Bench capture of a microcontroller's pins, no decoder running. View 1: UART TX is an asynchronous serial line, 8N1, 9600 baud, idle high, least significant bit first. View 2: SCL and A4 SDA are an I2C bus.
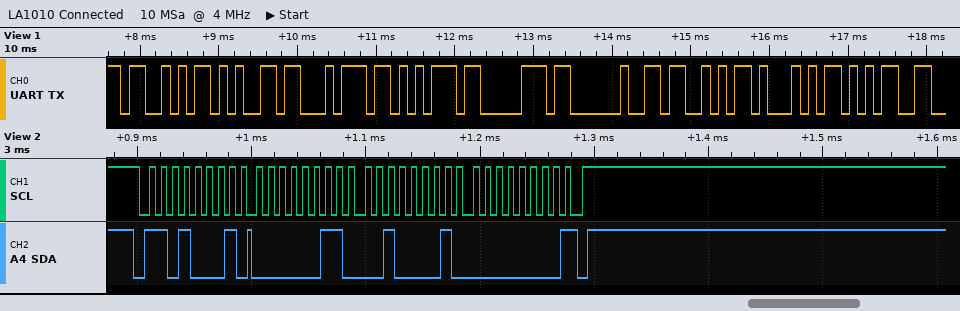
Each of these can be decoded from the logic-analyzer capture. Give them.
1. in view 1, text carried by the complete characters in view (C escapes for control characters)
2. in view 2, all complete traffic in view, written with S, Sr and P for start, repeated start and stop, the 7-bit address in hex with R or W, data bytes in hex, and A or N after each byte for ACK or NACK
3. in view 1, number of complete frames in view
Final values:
"Setup SQ5"
S 68R A 03 A 21 A 00 N P
9
